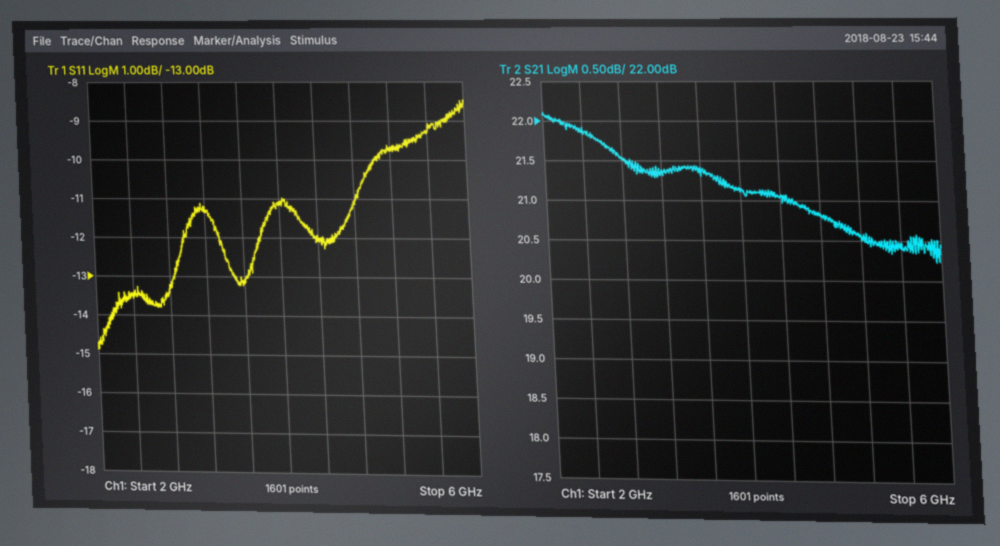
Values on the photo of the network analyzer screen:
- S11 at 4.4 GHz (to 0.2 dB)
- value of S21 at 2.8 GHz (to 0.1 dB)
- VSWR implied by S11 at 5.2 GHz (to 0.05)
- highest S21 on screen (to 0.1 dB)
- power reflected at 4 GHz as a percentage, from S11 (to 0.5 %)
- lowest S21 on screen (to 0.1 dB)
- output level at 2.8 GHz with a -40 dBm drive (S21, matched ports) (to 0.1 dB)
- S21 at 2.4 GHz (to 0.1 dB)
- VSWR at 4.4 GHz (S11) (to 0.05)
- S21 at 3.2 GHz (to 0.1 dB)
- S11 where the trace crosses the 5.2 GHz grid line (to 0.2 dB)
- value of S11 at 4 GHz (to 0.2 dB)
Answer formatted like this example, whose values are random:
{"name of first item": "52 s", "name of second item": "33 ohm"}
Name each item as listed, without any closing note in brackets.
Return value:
{"S11 at 4.4 GHz": "-12.0 dB", "value of S21 at 2.8 GHz": "21.5 dB", "VSWR implied by S11 at 5.2 GHz": "1.95", "highest S21 on screen": "22.1 dB", "power reflected at 4 GHz as a percentage, from S11": "7.5 %", "lowest S21 on screen": "20.2 dB", "output level at 2.8 GHz with a -40 dBm drive (S21, matched ports)": "-18.5 dBm", "S21 at 2.4 GHz": "21.9 dB", "VSWR at 4.4 GHz (S11)": "1.65", "S21 at 3.2 GHz": "21.4 dB", "S11 where the trace crosses the 5.2 GHz grid line": "-9.8 dB", "value of S11 at 4 GHz": "-11.2 dB"}
